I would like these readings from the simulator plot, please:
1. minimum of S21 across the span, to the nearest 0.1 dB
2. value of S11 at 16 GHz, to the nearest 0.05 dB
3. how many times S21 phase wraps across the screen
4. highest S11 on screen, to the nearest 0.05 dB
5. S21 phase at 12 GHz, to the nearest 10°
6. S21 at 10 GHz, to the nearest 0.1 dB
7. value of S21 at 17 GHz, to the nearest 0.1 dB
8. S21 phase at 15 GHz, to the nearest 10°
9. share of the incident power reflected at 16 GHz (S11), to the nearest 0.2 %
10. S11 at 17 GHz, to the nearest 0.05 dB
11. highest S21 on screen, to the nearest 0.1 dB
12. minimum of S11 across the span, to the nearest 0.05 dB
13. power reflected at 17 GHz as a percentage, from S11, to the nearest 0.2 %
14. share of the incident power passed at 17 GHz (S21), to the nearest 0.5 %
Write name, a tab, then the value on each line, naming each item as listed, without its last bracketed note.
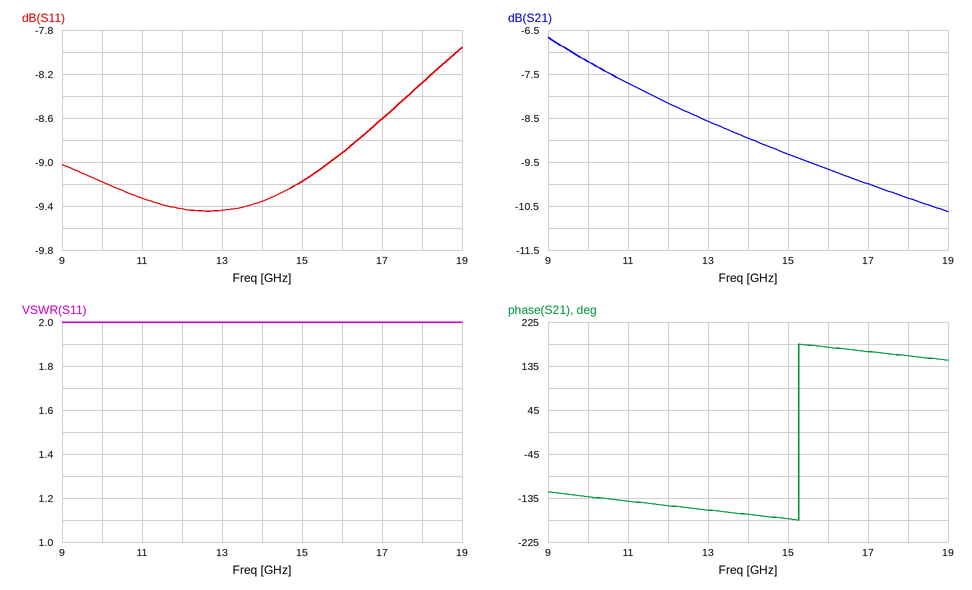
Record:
minimum of S21 across the span, to the nearest 0.1 dB	-10.6 dB
value of S11 at 16 GHz, to the nearest 0.05 dB	-8.90 dB
how many times S21 phase wraps across the screen	1
highest S11 on screen, to the nearest 0.05 dB	-7.95 dB
S21 phase at 12 GHz, to the nearest 10°	-150°
S21 at 10 GHz, to the nearest 0.1 dB	-7.2 dB
value of S21 at 17 GHz, to the nearest 0.1 dB	-10.0 dB
S21 phase at 15 GHz, to the nearest 10°	-180°
share of the incident power reflected at 16 GHz (S11), to the nearest 0.2 %	12.8 %
S11 at 17 GHz, to the nearest 0.05 dB	-8.60 dB
highest S21 on screen, to the nearest 0.1 dB	-6.7 dB
minimum of S11 across the span, to the nearest 0.05 dB	-9.45 dB
power reflected at 17 GHz as a percentage, from S11, to the nearest 0.2 %	13.8 %
share of the incident power passed at 17 GHz (S21), to the nearest 0.5 %	10.0 %
